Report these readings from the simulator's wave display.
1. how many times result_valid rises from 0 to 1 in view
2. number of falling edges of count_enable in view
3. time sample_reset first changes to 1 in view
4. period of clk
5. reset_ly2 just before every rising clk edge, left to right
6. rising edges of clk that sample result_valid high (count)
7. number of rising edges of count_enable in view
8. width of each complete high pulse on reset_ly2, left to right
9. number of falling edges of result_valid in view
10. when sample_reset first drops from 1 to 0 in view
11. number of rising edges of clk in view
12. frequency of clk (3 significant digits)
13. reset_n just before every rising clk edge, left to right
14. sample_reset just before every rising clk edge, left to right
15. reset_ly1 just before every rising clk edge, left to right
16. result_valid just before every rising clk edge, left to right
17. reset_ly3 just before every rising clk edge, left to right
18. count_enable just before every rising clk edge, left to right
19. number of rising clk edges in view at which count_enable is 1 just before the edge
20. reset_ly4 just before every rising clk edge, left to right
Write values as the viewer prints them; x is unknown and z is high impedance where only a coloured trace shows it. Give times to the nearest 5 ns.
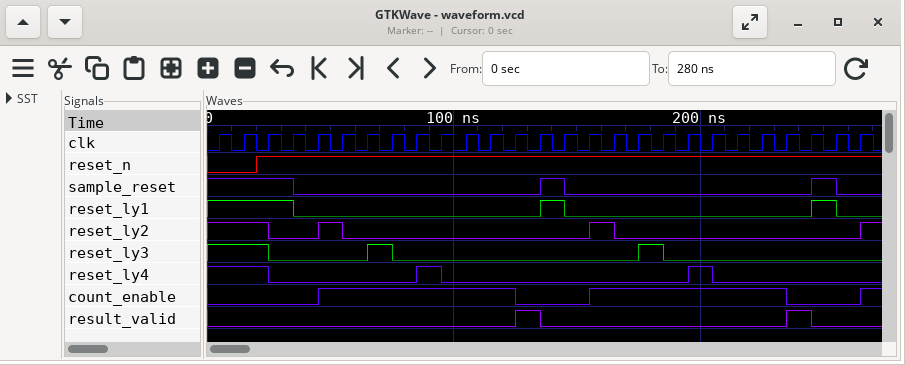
2
2
135 ns
10 ns
1 1 1 0 0 1 0 0 0 0 0 0 0 0 0 0 1 0 0 0 0 0 0 0 0 0 0
2
3
10 ns, 10 ns
2
35 ns
27
100 MHz
0 0 1 1 1 1 1 1 1 1 1 1 1 1 1 1 1 1 1 1 1 1 1 1 1 1 1
1 1 1 1 0 0 0 0 0 0 0 0 0 0 1 0 0 0 0 0 0 0 0 0 0 1 0
1 1 1 1 0 0 0 0 0 0 0 0 0 0 1 0 0 0 0 0 0 0 0 0 0 1 0
0 0 0 0 0 0 0 0 0 0 0 0 0 1 0 0 0 0 0 0 0 0 0 0 1 0 0
1 1 1 0 0 0 0 1 0 0 0 0 0 0 0 0 0 0 1 0 0 0 0 0 0 0 0
0 0 0 0 0 1 1 1 1 1 1 1 1 0 0 0 1 1 1 1 1 1 1 1 0 0 0
16
1 1 1 0 0 0 0 0 0 1 0 0 0 0 0 0 0 0 0 0 1 0 0 0 0 0 0
